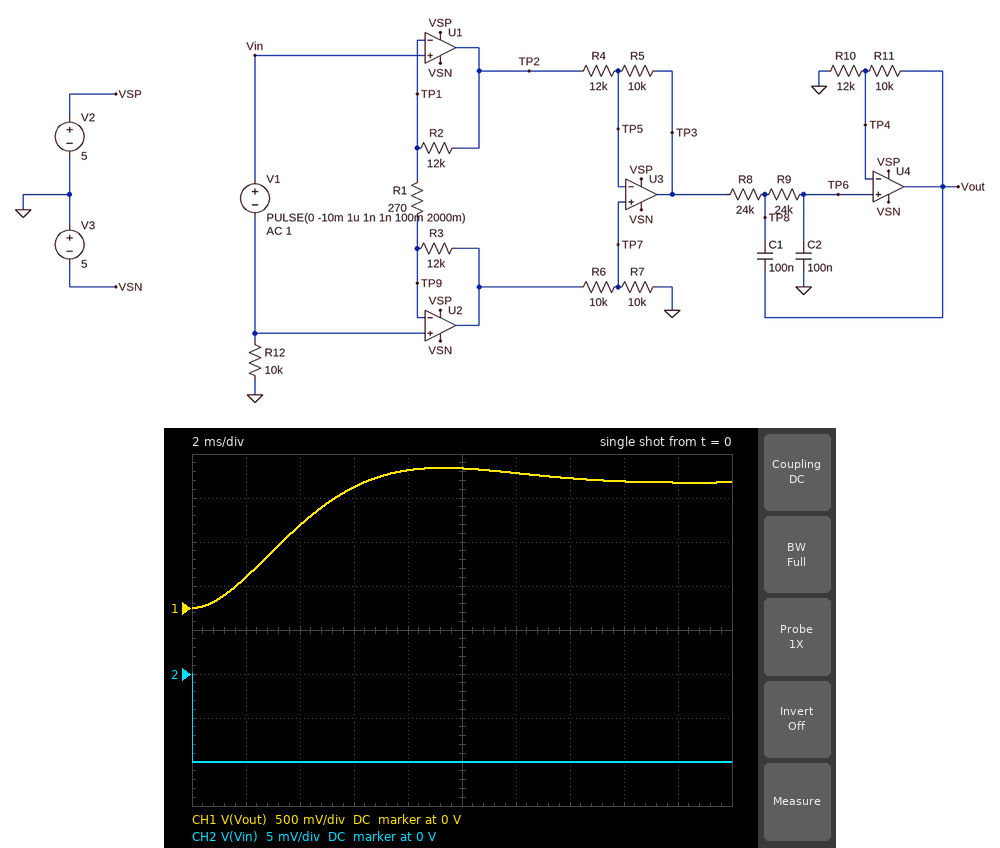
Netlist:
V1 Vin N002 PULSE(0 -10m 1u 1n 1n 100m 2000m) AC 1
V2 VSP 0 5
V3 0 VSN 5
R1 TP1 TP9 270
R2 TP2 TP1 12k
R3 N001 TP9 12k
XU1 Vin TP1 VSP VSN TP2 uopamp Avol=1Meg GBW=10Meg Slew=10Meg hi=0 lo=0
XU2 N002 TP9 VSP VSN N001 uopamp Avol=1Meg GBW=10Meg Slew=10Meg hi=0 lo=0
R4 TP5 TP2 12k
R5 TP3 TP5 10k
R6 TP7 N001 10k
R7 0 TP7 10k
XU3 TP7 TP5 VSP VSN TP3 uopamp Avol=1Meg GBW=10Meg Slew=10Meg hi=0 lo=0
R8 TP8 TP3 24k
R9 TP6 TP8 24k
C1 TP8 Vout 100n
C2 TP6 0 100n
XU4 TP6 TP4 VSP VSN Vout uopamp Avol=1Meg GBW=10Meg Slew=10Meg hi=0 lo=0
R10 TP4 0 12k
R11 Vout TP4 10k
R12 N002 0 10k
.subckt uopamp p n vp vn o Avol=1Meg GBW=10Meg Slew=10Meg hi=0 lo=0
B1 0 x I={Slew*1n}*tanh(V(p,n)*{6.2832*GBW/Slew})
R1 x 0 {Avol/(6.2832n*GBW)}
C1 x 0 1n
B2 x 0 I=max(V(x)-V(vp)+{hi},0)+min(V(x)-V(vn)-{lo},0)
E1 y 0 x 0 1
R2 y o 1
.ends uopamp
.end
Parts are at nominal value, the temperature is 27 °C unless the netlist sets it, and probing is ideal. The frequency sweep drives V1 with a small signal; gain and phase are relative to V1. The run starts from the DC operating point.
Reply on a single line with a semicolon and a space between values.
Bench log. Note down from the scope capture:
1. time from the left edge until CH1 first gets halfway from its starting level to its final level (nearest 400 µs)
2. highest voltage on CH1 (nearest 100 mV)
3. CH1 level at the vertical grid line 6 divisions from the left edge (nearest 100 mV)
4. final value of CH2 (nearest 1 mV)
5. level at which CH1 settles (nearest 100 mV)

3.2 ms; 1.6 V; 1.5 V; -10 mV; 1.4 V
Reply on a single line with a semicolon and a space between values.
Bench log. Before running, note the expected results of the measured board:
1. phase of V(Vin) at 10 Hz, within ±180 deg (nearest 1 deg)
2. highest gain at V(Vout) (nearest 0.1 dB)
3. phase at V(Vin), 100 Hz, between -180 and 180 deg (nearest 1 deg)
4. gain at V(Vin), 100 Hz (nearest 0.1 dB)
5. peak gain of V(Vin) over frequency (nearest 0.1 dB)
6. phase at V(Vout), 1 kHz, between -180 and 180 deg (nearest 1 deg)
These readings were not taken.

0 deg; 43.6 dB; 0 deg; 0 dB; 0 dB; 4 deg
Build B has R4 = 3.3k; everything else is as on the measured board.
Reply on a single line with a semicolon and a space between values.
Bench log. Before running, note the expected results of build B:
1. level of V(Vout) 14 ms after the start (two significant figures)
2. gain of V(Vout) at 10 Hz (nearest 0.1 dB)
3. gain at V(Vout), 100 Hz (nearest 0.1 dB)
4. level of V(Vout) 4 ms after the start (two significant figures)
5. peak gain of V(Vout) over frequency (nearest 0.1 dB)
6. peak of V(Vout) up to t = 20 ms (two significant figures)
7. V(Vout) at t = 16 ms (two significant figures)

4.3 V; 52.5 dB; 45.7 dB; 2.7 V; 52.9 dB; 4.6 V; 4.2 V
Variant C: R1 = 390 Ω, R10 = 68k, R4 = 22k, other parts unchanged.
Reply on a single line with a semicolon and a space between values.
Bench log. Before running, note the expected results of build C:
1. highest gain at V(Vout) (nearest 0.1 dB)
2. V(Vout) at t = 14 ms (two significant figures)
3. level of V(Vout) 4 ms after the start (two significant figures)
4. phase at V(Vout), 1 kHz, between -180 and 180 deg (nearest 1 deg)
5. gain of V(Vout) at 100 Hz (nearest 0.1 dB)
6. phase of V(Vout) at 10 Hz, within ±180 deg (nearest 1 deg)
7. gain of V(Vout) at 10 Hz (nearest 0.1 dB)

32.5 dB; 420 mV; 220 mV; 7 deg; 22.8 dB; 164 deg; 32.4 dB
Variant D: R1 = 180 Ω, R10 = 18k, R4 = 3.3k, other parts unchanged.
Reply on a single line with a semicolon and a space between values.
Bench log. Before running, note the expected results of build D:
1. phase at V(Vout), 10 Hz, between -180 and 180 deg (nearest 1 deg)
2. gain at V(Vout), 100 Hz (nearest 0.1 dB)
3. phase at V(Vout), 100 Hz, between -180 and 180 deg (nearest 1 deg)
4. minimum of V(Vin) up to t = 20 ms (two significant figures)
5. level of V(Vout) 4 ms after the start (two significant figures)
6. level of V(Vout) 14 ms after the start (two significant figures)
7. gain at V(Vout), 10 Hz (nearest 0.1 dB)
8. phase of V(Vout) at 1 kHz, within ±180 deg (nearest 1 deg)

167 deg; 46.4 dB; 60 deg; -10 mV; 3.1 V; 5.0 V; 54.4 dB; 5 deg
